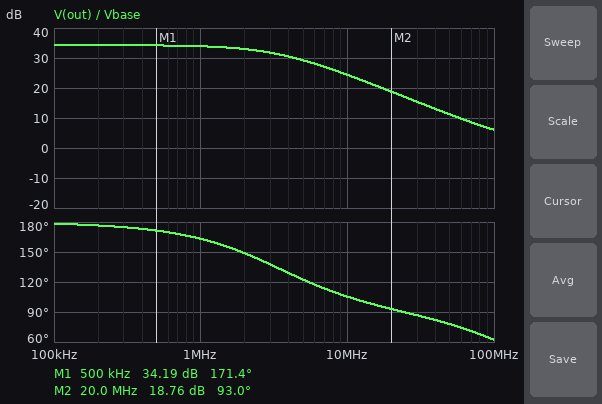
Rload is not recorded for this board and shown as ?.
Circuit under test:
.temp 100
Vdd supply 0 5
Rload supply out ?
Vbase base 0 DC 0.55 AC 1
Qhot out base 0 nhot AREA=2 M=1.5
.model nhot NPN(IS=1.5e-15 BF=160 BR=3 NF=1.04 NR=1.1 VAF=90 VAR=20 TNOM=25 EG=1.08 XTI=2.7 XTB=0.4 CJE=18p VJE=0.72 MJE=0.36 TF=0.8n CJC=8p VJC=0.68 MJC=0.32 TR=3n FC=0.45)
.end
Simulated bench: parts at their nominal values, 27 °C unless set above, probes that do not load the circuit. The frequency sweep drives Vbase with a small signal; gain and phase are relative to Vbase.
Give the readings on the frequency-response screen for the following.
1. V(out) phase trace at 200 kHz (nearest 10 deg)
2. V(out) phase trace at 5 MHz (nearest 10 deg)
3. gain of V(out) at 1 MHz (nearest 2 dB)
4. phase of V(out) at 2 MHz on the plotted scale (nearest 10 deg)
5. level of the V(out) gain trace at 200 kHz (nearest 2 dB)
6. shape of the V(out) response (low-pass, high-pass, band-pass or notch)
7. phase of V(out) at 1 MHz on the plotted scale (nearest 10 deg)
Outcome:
180 deg
120 deg
34 dB
150 deg
34 dB
low-pass
160 deg
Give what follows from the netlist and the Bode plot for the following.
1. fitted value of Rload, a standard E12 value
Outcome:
3.3 kΩ
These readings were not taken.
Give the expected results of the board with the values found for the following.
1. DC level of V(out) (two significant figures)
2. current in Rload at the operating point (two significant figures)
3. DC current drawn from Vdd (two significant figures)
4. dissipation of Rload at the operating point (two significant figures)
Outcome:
3.2 V
540 µA
540 µA
950 µW
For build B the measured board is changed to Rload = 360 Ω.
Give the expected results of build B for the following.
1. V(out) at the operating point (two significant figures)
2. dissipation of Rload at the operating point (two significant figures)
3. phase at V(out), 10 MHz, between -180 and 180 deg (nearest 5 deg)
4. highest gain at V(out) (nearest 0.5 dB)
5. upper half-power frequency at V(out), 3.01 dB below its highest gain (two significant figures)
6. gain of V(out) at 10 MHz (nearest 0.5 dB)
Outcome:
4.8 V
110 µW
160 deg
15.5 dB
36 MHz
15.0 dB
